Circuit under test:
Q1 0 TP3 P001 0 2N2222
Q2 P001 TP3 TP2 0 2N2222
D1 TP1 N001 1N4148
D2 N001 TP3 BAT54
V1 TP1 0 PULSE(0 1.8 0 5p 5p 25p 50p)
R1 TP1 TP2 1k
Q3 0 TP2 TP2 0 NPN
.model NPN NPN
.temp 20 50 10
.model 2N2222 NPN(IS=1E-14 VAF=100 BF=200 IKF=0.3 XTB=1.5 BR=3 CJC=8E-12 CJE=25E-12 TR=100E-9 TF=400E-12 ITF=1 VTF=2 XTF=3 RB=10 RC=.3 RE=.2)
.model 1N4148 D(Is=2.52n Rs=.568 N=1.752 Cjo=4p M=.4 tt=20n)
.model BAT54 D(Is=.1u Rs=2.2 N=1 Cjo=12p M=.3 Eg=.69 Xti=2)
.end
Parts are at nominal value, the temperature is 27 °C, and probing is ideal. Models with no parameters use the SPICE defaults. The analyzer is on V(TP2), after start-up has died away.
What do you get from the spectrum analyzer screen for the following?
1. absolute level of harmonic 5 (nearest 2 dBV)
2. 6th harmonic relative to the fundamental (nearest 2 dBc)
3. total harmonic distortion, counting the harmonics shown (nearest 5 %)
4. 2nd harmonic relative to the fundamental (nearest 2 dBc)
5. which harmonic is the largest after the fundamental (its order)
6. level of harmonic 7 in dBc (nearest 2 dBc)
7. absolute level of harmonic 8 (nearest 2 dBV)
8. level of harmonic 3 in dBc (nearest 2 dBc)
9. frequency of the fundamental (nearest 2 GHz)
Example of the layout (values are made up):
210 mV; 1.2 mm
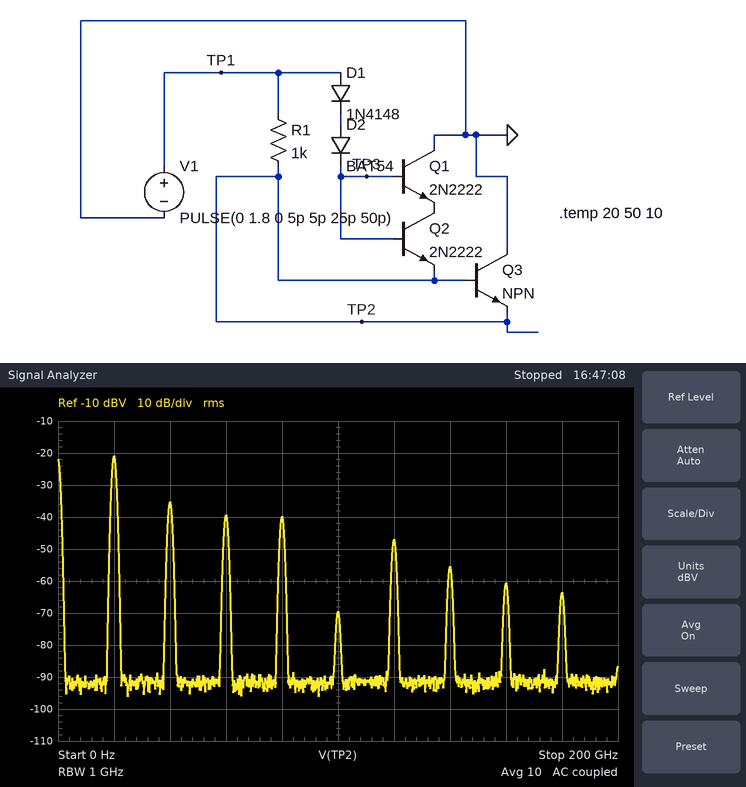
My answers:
-70 dBV; -26 dBc; 25 %; -14 dBc; 2; -34 dBc; -60 dBV; -18 dBc; 20 GHz
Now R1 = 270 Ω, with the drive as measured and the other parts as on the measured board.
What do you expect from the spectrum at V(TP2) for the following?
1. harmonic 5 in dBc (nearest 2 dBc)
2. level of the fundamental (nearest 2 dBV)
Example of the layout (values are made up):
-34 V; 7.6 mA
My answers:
-46 dBc; -20 dBV
